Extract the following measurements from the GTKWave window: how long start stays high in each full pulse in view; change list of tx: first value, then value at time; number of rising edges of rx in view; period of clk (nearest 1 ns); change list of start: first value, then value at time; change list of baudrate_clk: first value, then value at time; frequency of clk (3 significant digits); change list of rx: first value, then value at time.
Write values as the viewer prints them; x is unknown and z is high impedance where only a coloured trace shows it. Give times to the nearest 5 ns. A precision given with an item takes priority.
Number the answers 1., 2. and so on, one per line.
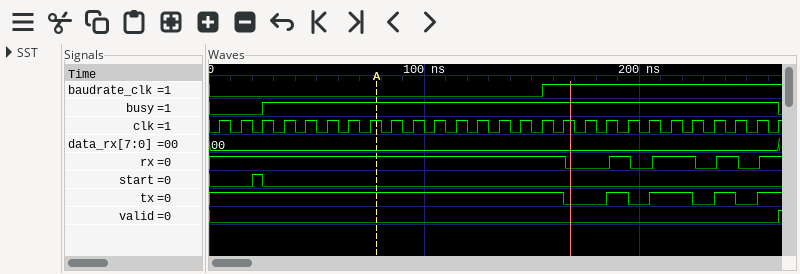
1. 5 ns
2. 1, 0 at 165 ns, 1 at 185 ns, 0 at 195 ns, 1 at 205 ns, 0 at 225 ns, 1 at 235 ns, 0 at 245 ns, 1 at 255 ns
3. 4
4. 10 ns
5. 0, 1 at 20 ns, 0 at 25 ns
6. 0, 1 at 155 ns
7. 100 MHz
8. 1, 0 at 165 ns, 1 at 185 ns, 0 at 195 ns, 1 at 205 ns, 0 at 225 ns, 1 at 235 ns, 0 at 245 ns, 1 at 255 ns
